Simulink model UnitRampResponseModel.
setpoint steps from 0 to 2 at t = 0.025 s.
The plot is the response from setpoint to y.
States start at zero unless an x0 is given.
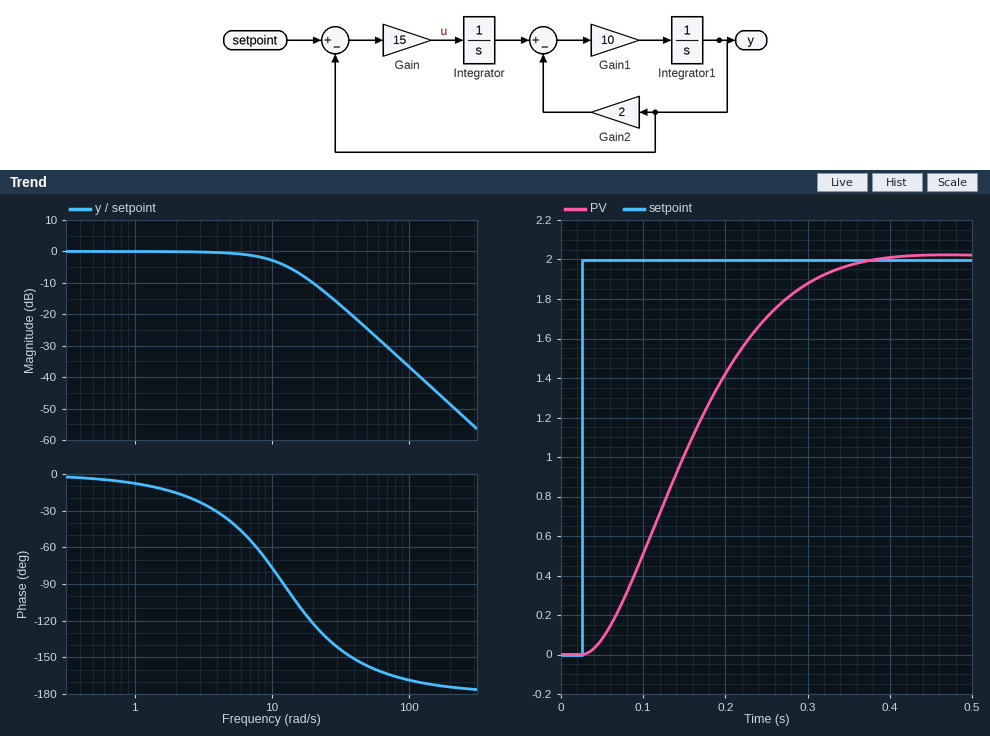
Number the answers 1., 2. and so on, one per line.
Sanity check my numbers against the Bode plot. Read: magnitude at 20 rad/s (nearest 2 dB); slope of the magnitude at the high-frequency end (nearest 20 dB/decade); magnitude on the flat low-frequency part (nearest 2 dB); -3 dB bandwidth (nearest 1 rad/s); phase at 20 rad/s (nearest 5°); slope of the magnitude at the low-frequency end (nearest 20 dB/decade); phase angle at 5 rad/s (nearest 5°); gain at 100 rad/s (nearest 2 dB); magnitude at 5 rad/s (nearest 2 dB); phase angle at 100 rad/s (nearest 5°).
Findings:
1. -10 dB
2. -40 dB/decade
3. 0 dB
4. 10 rad/s
5. -120°
6. 0 dB/decade
7. -40°
8. -36 dB
9. 0 dB
10. -170°
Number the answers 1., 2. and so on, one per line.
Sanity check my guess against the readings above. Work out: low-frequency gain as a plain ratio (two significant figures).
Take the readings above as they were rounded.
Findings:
1. 1.0
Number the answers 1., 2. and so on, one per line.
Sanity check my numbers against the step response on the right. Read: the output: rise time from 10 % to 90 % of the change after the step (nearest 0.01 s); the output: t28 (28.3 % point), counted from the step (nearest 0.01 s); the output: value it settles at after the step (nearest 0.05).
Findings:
1. 0.21 s
2. 0.08 s
3. 2.00
